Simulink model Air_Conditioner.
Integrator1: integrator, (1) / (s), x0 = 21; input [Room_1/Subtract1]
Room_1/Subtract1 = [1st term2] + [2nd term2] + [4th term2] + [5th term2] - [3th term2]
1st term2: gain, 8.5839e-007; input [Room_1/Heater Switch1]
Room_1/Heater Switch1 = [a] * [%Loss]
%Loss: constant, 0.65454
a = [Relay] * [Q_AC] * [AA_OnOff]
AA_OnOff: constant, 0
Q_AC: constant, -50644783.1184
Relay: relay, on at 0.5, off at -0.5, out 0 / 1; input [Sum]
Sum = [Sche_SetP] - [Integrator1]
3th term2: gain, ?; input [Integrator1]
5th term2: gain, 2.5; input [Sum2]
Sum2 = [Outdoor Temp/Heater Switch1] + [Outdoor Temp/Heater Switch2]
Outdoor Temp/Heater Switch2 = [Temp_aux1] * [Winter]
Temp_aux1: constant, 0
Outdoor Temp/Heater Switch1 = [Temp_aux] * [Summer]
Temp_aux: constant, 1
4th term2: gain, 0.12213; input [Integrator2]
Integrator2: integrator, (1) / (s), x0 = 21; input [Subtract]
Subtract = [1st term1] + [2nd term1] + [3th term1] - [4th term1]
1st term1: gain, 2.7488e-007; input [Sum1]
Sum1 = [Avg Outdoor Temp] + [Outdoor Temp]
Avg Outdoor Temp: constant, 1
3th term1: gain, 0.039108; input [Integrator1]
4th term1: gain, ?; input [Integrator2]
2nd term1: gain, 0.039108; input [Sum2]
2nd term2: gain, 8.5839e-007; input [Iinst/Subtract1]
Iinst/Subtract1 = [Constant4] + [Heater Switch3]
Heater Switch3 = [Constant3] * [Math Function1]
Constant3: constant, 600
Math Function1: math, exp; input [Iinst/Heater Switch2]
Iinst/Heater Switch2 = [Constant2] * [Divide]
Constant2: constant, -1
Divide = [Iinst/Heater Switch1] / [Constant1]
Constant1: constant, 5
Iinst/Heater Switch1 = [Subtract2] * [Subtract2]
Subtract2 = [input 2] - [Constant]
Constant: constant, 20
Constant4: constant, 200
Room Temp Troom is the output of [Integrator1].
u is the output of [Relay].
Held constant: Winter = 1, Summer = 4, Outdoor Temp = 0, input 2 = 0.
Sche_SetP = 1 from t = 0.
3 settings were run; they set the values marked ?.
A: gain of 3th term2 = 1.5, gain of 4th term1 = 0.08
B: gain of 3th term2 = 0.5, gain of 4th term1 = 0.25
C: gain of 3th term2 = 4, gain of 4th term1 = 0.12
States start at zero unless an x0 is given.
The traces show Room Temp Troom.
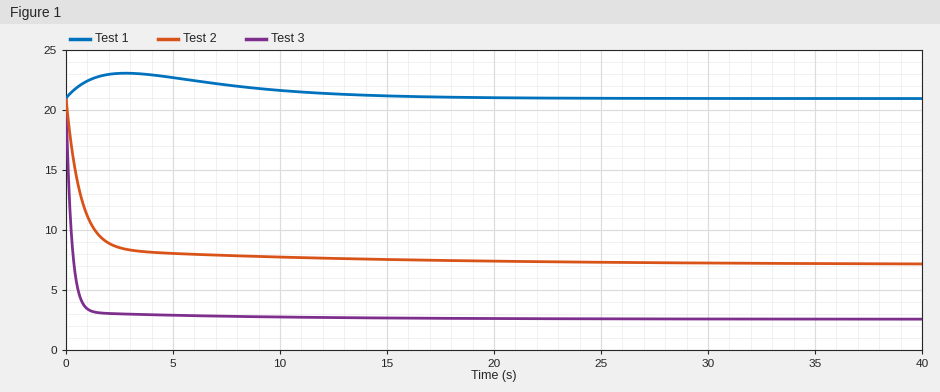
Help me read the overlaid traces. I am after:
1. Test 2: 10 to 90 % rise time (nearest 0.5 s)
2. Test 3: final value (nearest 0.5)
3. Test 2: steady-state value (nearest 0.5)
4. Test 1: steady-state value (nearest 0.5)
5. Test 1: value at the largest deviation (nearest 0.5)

2.5 s
2.5
7.0
21.0
23.0
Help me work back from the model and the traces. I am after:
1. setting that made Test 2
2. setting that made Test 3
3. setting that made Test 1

A
C
B
